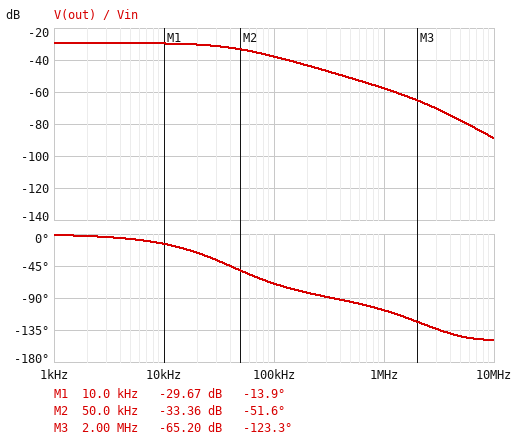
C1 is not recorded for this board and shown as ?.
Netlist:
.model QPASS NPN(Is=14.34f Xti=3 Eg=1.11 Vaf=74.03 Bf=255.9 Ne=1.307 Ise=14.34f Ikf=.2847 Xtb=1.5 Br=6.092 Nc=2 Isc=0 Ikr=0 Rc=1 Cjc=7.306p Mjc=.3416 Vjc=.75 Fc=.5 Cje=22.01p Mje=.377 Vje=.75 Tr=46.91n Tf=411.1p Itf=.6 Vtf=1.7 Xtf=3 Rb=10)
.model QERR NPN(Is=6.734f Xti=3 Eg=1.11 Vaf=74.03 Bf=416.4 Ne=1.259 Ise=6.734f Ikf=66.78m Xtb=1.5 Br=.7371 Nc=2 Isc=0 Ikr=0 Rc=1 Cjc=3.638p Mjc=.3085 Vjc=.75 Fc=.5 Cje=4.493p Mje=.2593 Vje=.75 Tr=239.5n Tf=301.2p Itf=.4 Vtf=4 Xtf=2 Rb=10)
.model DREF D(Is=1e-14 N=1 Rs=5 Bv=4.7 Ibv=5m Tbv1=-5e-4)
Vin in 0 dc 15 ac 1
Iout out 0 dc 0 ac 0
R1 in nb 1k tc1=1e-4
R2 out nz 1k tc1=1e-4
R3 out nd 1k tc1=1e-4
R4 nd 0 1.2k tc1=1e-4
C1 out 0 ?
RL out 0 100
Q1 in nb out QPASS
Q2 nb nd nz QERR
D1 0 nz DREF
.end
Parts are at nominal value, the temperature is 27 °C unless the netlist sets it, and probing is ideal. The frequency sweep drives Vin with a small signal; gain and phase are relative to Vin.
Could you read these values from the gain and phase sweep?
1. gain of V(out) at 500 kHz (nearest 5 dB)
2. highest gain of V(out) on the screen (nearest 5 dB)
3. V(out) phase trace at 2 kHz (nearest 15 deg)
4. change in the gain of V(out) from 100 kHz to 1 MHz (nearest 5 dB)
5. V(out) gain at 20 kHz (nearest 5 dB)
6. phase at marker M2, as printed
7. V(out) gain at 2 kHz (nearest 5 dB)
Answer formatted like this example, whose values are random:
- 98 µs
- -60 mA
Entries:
- -50 dB
- -30 dB
- 0 deg
- -20 dB
- -30 dB
- -51.6 deg
- -30 dB
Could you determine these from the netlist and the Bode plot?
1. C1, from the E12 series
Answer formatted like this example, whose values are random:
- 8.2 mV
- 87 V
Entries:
- 15 µF
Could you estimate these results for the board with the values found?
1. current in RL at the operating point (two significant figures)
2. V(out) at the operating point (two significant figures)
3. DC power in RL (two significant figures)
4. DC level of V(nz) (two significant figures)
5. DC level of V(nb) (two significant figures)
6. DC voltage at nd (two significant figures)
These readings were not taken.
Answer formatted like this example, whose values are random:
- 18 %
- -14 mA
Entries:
- 100 mA
- 10 V
- 1.0 W
- 4.8 V
- 11 V
- 5.5 V
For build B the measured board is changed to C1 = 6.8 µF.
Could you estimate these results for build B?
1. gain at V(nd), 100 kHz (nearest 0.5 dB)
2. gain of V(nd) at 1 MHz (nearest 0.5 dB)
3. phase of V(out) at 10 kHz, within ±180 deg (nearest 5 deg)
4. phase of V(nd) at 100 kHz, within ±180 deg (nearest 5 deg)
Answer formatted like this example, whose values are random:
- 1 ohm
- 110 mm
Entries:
- -39.5 dB
- -59.5 dB
- -5 deg
- -50 deg
